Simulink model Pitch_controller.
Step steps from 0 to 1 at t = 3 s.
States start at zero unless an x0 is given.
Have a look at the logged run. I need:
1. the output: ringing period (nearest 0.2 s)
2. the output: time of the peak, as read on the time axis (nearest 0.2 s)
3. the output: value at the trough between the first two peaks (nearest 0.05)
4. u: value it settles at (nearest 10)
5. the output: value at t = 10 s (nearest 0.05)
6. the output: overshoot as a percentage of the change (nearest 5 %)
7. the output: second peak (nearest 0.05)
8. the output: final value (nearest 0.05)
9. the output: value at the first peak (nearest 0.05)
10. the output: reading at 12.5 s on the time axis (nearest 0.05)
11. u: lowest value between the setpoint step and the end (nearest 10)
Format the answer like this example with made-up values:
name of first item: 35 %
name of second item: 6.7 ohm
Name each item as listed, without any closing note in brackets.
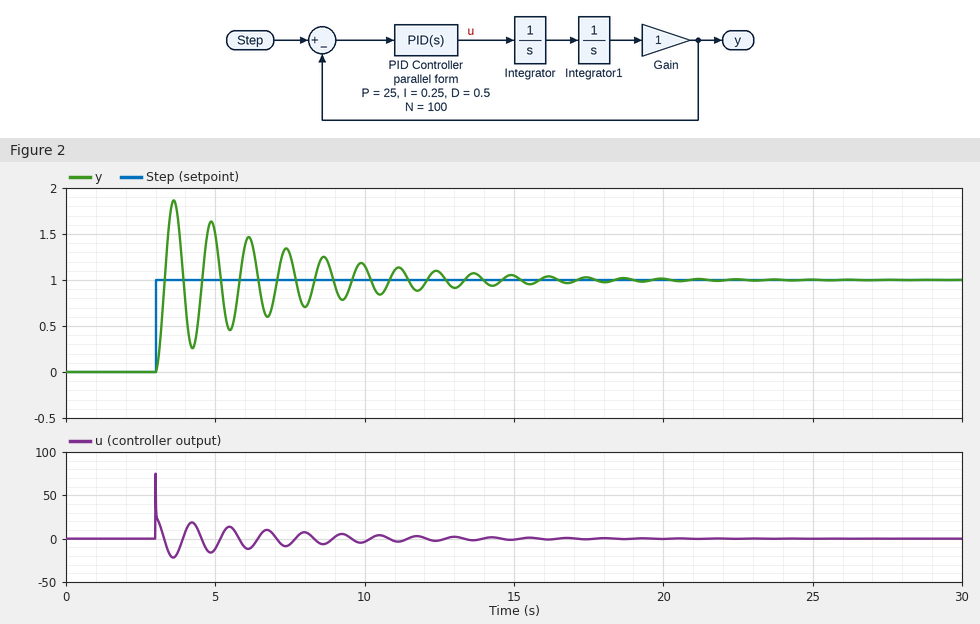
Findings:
the output: ringing period: 1.2 s
the output: time of the peak, as read on the time axis: 3.6 s
the output: value at the trough between the first two peaks: 0.25
u: value it settles at: 0
the output: value at t = 10 s: 1.15
the output: overshoot as a percentage of the change: 85 %
the output: second peak: 1.65
the output: final value: 1.00
the output: value at the first peak: 1.85
the output: reading at 12.5 s on the time axis: 1.10
u: lowest value between the setpoint step and the end: -20
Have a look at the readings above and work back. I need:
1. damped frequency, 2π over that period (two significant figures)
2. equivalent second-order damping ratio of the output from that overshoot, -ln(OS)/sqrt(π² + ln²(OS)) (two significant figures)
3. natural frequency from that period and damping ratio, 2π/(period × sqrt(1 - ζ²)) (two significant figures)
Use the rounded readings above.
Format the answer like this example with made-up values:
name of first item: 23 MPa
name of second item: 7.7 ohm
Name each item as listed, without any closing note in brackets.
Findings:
damped frequency, 2π over that period: 5.2 rad/s
equivalent second-order damping ratio of the output from that overshoot, -ln(OS)/sqrt(π² + ln²(OS)): 0.052
natural frequency from that period and damping ratio, 2π/(period × sqrt(1 - ζ²)): 5.2 rad/s
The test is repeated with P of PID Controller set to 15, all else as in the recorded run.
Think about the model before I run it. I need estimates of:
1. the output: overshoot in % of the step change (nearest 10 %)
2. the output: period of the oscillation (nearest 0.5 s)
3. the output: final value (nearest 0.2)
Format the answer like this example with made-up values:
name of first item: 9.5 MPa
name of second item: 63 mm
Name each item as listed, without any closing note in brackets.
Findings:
the output: overshoot in % of the step change: 80 %
the output: period of the oscillation: 1.5 s
the output: final value: 1.0
